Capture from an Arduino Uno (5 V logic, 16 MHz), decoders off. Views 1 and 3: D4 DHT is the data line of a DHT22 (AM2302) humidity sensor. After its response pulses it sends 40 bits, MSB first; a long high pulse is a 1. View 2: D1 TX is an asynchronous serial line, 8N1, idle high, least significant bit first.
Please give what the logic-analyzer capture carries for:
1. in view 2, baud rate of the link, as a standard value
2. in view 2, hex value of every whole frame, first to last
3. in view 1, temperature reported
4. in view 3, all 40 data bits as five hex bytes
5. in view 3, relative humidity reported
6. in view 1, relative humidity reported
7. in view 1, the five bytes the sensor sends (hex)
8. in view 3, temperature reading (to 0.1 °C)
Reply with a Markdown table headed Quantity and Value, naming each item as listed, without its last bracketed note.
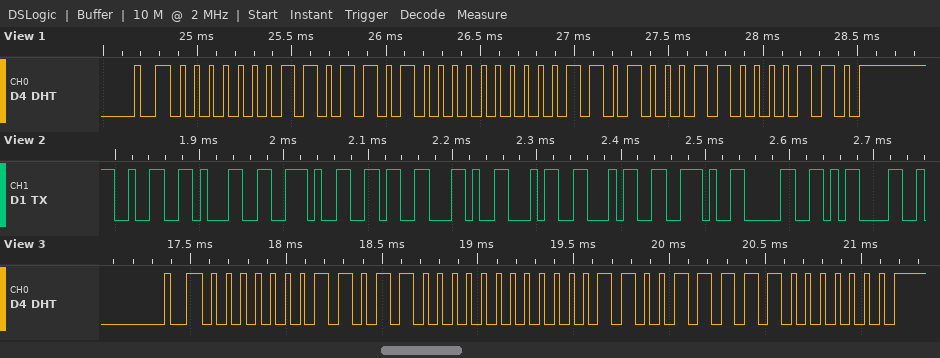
| Quantity | Value |
|---|---|
| in view 2, baud rate of the link, as a standard value | 115200 baud |
| in view 2, hex value of every whole frame, first to last | 32 31 2E 36 2C 34 34 2E 30 0D |
| in view 1, temperature reported | 20.9 °C |
| in view 3, all 40 data bits as five hex bytes | 01 B0 00 CF 80 |
| in view 3, relative humidity reported | 43.2 % |
| in view 1, relative humidity reported | 43.6 % |
| in view 1, the five bytes the sensor sends | 01 B4 00 D1 86 |
| in view 3, temperature reading | 20.7 °C |
